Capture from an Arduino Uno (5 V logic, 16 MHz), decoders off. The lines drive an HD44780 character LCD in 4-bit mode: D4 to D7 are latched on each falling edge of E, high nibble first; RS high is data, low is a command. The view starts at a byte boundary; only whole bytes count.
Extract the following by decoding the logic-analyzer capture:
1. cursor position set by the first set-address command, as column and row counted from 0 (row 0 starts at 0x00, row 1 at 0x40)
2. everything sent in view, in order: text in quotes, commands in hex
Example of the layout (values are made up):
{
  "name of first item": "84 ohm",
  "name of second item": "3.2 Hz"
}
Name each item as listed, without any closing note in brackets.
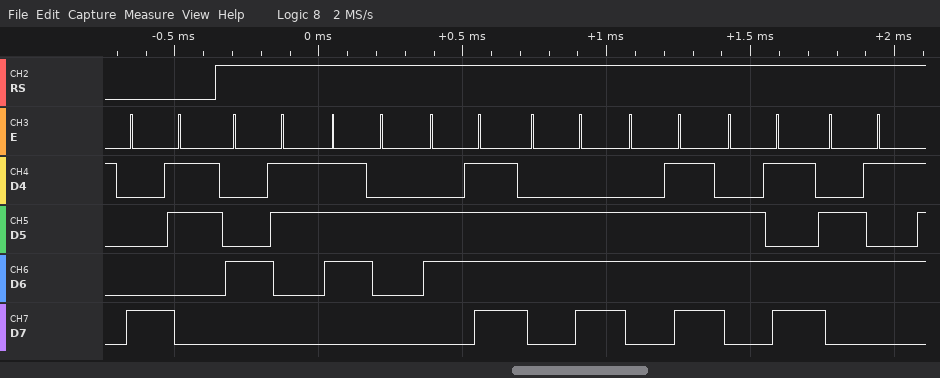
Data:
{
  "cursor position set by the first set-address command, as column and row counted from 0": "column 3, row 0",
  "everything sent in view, in order: text in quotes, commands in hex": "0x83 \"Cronome\""
}
